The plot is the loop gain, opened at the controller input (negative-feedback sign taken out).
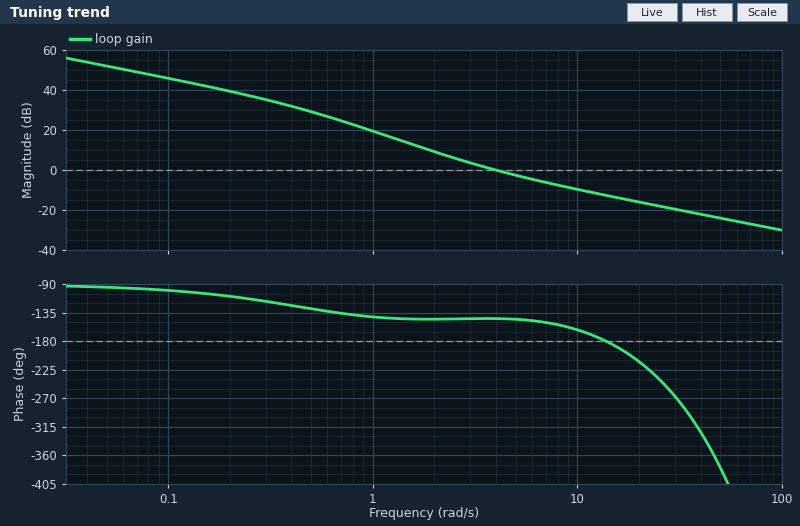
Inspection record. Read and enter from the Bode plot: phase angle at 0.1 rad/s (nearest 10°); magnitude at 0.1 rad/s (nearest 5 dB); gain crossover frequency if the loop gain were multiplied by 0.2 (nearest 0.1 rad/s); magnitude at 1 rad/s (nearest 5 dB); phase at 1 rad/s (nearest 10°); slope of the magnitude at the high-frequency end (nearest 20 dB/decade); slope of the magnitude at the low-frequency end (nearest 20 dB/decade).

-100°
45 dB
1.4 rad/s
20 dB
-140°
-20 dB/decade
-20 dB/decade
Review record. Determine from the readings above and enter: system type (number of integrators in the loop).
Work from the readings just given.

1
